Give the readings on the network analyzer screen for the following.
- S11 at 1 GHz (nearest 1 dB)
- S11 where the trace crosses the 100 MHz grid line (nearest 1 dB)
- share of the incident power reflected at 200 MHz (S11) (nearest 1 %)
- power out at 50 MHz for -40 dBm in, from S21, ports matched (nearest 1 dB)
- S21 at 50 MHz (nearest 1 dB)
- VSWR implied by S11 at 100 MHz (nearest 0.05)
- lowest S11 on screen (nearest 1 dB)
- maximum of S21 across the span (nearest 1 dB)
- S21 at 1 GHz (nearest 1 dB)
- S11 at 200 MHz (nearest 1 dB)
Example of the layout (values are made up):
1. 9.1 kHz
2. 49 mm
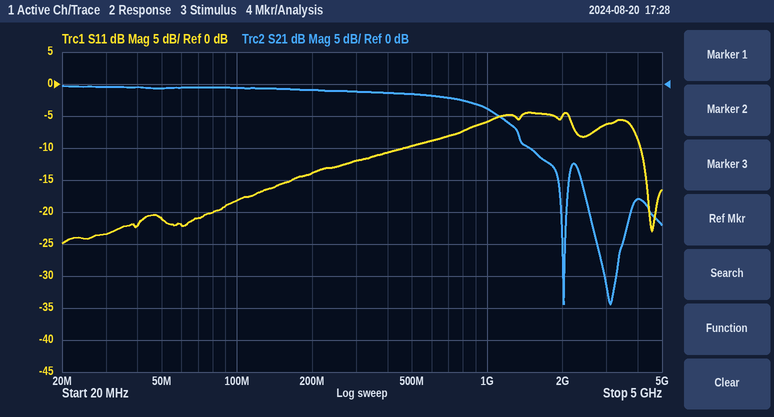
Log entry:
1. -6 dB
2. -18 dB
3. 4 %
4. -41 dBm
5. -1 dB
6. 1.30
7. -25 dB
8. 0 dB
9. -4 dB
10. -14 dB
